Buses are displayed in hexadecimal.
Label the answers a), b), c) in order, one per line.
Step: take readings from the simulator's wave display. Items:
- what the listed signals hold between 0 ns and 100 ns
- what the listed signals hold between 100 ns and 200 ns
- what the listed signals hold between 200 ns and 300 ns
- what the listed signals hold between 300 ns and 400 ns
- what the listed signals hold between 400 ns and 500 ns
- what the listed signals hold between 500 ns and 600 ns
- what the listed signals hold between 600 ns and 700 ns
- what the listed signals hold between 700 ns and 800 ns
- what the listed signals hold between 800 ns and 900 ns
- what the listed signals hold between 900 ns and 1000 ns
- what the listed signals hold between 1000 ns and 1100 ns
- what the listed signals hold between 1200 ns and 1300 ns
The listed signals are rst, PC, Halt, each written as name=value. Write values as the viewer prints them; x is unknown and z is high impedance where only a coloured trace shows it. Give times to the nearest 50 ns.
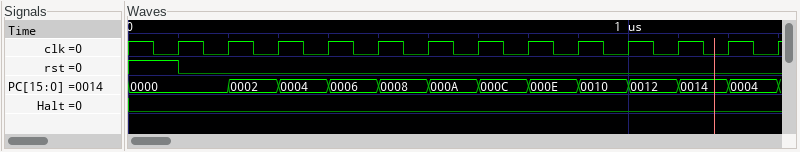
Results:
a) rst=1, PC=0000, Halt=0
b) rst=0, PC=0000, Halt=0
c) rst=0, PC=0002, Halt=0
d) rst=0, PC=0004, Halt=0
e) rst=0, PC=0006, Halt=0
f) rst=0, PC=0008, Halt=0
g) rst=0, PC=000A, Halt=0
h) rst=0, PC=000C, Halt=0
i) rst=0, PC=000E, Halt=0
j) rst=0, PC=0010, Halt=0
k) rst=0, PC=0012, Halt=0
l) rst=0, PC=0004, Halt=0
